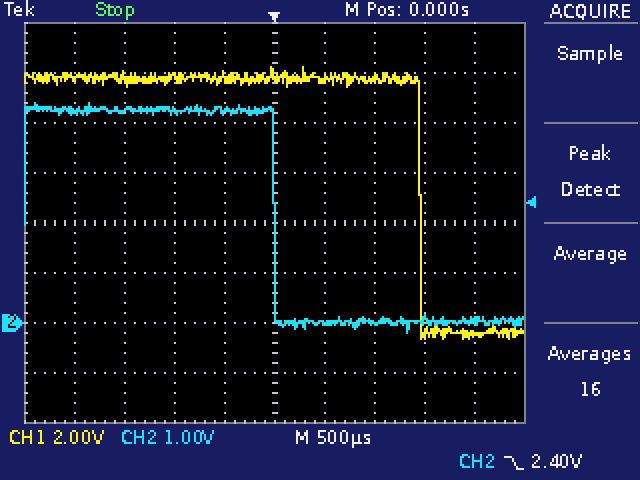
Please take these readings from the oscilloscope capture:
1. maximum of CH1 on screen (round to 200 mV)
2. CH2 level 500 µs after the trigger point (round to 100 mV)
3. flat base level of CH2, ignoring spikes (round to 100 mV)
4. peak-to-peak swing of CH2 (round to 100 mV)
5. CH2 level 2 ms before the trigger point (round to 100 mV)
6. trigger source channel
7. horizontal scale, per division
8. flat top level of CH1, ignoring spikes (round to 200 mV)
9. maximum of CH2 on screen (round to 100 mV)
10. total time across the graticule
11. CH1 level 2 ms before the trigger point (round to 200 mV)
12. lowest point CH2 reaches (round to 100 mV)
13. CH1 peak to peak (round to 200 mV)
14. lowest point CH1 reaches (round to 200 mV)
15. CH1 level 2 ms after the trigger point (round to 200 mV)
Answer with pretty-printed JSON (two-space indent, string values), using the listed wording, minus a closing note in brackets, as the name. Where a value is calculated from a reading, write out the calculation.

{
  "maximum of CH1 on screen": "10.2 V",
  "CH2 level 500 µs after the trigger point": "0.0 V",
  "flat base level of CH2, ignoring spikes": "0.0 V",
  "peak-to-peak swing of CH2": "4.4 V − (-200 mV) = 4.6 V",
  "CH2 level 2 ms before the trigger point": "4.2 V",
  "trigger source channel": "CH2",
  "horizontal scale, per division": "500 µs",
  "flat top level of CH1, ignoring spikes": "9.8 V",
  "maximum of CH2 on screen": "4.4 V",
  "total time across the graticule": "5 ms",
  "CH1 level 2 ms before the trigger point": "9.8 V",
  "lowest point CH2 reaches": "-200 mV",
  "CH1 peak to peak": "10.2 V − (-600 mV) = 10.8 V",
  "lowest point CH1 reaches": "-600 mV",
  "CH1 level 2 ms after the trigger point": "-400 mV"
}
